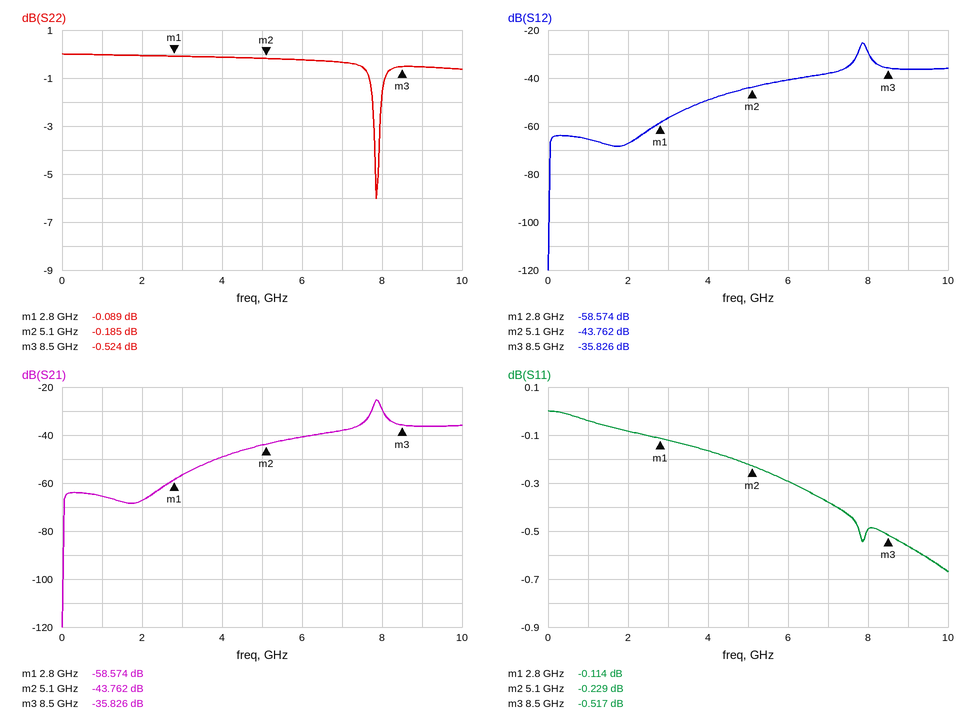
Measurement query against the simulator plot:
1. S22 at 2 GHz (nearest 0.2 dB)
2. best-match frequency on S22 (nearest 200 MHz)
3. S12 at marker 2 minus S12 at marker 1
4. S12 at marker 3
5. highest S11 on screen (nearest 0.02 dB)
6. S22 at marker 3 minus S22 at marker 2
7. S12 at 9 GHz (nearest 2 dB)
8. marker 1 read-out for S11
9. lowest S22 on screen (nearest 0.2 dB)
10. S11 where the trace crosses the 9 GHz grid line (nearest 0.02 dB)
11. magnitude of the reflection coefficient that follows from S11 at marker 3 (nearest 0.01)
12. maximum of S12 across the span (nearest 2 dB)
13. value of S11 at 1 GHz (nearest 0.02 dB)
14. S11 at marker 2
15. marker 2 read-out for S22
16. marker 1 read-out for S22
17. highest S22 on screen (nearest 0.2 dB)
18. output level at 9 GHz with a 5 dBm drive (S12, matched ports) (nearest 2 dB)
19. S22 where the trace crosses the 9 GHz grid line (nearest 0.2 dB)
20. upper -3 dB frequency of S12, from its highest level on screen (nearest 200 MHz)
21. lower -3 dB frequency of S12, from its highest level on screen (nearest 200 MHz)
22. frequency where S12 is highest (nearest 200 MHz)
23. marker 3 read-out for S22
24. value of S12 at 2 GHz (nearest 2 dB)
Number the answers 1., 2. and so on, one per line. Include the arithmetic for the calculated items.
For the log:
1. 0.0 dB
2. 7.8 GHz
3. -43.762 − (-58.574) = 14.812 dB
4. -35.826 dB
5. 0.00 dB
6. -0.524 − (-0.185) = -0.339 dB
7. -36 dB
8. -0.114 dB
9. -6.0 dB
10. -0.56 dB
11. 10^(-0.517/20) ≈ 0.94
12. -26 dB
13. -0.04 dB
14. -0.229 dB
15. -0.185 dB
16. -0.089 dB
17. 0.0 dB
18. 5 dBm + (-36 dB) = -32 dBm
19. -0.6 dB
20. 8.0 GHz
21. 7.8 GHz
22. 7.8 GHz
23. -0.524 dB
24. -68 dB
